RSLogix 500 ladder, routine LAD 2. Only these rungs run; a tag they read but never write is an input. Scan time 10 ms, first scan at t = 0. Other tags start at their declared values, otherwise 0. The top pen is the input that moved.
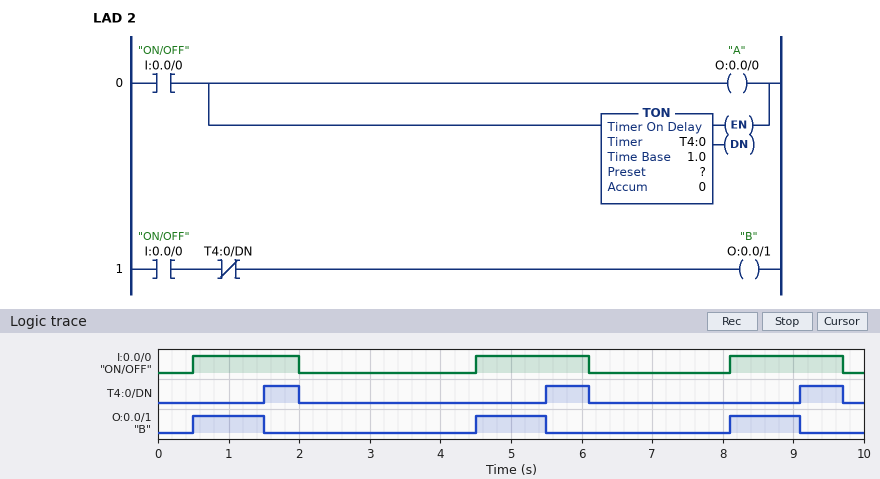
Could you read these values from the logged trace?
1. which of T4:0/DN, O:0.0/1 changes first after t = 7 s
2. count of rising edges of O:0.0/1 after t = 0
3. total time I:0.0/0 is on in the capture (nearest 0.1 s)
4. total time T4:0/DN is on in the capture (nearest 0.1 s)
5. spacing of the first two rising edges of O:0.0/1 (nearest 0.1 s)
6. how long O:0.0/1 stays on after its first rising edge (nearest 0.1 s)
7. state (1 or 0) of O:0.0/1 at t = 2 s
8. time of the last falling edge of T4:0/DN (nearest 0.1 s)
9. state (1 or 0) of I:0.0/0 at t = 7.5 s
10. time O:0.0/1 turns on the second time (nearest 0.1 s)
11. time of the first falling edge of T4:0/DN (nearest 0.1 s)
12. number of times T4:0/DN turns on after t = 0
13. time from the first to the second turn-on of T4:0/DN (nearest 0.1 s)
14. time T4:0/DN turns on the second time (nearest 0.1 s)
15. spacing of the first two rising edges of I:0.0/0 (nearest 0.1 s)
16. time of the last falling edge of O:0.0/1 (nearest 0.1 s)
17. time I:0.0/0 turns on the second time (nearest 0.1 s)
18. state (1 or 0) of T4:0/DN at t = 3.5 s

O:0.0/1
3
4.7 s
1.7 s
4.0 s
1.0 s
0
9.7 s
0
4.5 s
2.0 s
3
4.0 s
5.5 s
4.0 s
9.1 s
4.5 s
0
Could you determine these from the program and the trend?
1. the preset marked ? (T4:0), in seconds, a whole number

1 s
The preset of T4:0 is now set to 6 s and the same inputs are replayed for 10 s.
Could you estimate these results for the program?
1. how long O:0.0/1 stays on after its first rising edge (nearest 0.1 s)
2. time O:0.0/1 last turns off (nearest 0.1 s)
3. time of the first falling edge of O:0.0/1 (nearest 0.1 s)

1.5 s
9.7 s
2.0 s
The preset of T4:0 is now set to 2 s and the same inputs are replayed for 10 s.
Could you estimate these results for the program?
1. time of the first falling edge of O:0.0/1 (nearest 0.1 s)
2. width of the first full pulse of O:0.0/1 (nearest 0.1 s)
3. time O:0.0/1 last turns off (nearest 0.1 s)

2.0 s
1.5 s
9.7 s
